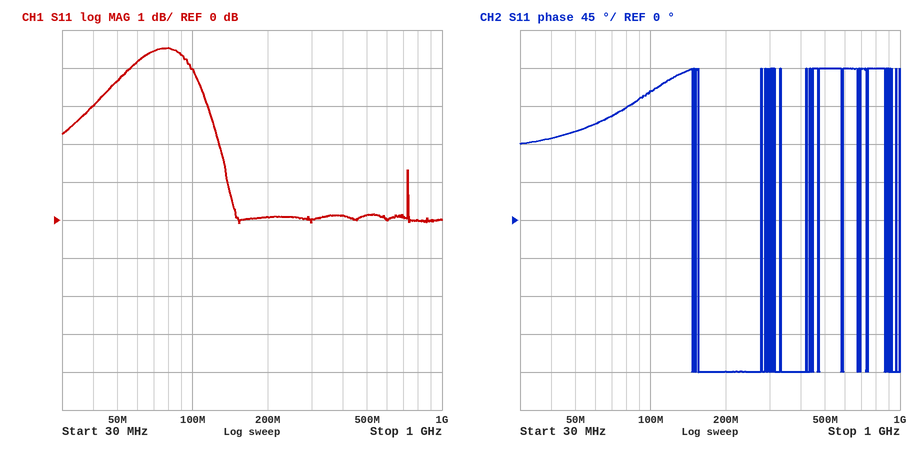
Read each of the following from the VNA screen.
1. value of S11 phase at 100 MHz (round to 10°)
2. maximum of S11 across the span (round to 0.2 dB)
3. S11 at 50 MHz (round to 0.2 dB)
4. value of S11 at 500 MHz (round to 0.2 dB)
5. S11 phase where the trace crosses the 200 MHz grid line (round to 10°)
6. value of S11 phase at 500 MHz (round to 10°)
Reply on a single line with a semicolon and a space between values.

150°; 4.6 dB; 3.6 dB; 0.2 dB; -180°; 180°
